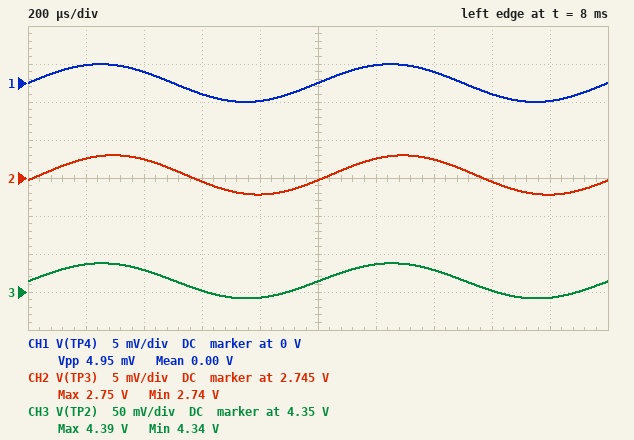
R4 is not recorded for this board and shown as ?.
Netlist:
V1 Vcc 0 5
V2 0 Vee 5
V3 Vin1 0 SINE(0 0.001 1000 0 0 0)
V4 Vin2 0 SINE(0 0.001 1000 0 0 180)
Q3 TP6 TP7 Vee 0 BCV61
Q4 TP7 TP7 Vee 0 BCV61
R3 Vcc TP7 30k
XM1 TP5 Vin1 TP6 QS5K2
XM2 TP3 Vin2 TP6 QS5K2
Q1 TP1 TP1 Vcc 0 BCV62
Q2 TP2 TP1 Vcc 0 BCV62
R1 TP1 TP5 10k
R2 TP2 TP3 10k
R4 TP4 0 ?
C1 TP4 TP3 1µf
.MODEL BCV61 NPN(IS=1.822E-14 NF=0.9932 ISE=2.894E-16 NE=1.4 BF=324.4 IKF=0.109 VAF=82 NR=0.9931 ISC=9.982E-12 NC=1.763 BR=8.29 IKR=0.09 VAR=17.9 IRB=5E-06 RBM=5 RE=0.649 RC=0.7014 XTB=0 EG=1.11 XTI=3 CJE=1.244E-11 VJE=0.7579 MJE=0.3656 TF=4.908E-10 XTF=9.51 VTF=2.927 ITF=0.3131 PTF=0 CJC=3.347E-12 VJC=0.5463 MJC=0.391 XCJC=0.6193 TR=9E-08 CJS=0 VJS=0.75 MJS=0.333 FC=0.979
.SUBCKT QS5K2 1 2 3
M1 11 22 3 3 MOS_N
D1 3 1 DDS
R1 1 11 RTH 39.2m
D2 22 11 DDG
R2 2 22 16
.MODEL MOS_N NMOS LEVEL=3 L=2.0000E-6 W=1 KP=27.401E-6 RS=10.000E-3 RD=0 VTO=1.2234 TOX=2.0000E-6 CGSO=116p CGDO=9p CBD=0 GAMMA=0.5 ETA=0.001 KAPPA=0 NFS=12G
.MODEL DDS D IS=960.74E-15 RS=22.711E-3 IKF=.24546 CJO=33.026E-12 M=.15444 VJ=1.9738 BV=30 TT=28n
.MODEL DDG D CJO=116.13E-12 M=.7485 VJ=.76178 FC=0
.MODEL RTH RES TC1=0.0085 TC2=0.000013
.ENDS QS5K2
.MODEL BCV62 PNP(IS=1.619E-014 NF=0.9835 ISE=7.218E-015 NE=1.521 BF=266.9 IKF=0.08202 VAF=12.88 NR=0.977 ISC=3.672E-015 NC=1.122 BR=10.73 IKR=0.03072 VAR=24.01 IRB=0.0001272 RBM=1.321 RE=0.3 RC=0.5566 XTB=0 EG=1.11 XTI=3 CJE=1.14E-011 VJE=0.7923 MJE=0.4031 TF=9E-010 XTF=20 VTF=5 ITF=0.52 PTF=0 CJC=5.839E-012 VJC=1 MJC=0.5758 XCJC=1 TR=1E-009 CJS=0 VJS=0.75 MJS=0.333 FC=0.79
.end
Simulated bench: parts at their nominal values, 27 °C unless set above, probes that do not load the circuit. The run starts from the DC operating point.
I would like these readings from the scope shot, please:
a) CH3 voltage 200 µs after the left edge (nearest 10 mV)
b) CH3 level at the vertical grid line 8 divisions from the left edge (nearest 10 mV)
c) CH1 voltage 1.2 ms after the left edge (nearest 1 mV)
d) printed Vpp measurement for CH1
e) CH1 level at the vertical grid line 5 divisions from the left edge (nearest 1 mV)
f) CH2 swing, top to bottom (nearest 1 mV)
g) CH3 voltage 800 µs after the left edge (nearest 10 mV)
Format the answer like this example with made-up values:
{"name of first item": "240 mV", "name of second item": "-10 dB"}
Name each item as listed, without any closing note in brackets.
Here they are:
{"CH3 voltage 200 µs after the left edge": "4.39 V", "CH3 level at the vertical grid line 8 divisions from the left edge": "4.35 V", "CH1 voltage 1.2 ms after the left edge": "2 mV", "printed Vpp measurement for CH1": "4.95 mV", "CH1 level at the vertical grid line 5 divisions from the left edge": "0 V", "CH2 swing, top to bottom": "5 mV", "CH3 voltage 800 µs after the left edge": "4.34 V"}
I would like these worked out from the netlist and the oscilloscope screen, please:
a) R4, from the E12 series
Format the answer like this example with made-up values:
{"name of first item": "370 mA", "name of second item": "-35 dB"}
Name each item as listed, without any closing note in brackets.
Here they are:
{"R4, from the E12 series": "560 Ω"}
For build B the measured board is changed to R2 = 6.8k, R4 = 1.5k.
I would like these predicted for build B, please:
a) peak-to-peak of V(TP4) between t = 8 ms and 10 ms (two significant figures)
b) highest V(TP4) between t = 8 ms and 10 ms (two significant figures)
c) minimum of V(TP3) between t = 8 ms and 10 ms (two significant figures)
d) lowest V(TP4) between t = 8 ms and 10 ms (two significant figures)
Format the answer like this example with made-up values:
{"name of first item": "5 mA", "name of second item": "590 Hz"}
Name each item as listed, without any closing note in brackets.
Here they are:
{"peak-to-peak of V(TP4) between t = 8 ms and 10 ms": "13 mV", "highest V(TP4) between t = 8 ms and 10 ms": "6.7 mV", "minimum of V(TP3) between t = 8 ms and 10 ms": "3.0 V", "lowest V(TP4) between t = 8 ms and 10 ms": "-6.7 mV"}
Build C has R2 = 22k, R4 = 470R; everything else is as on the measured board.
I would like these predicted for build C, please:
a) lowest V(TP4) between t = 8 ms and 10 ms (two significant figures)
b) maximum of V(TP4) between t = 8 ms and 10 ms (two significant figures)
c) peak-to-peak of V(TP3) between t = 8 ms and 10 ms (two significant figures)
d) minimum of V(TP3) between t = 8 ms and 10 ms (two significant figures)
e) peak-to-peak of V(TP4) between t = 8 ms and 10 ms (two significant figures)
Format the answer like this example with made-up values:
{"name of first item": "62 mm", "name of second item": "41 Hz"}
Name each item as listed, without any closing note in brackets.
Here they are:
{"lowest V(TP4) between t = 8 ms and 10 ms": "-1.2 mV", "maximum of V(TP4) between t = 8 ms and 10 ms": "1.2 mV", "peak-to-peak of V(TP3) between t = 8 ms and 10 ms": "2.6 mV", "minimum of V(TP3) between t = 8 ms and 10 ms": "1.5 V", "peak-to-peak of V(TP4) between t = 8 ms and 10 ms": "2.4 mV"}
